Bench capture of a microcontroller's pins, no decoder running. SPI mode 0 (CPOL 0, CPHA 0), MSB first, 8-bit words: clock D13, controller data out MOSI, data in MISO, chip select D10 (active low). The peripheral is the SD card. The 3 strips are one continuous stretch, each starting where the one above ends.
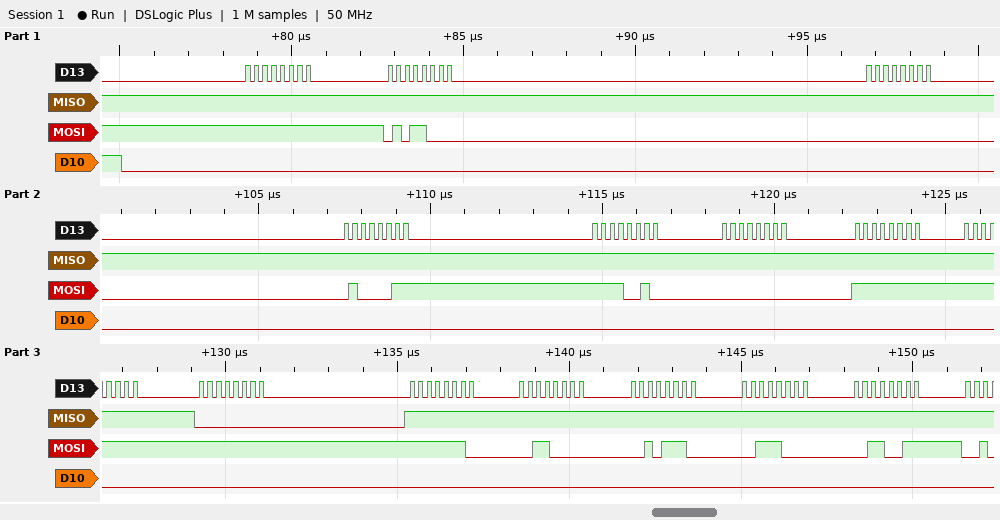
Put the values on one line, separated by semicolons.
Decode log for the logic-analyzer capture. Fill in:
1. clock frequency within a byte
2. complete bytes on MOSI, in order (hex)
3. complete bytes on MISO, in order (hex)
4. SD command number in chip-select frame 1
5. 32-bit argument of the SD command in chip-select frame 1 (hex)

4 MHz; FF 58 00 43 F2 00 FF FF FF FE 30 2E 38 33; FF FF FF FF FF FF FF FF 00 FF FF FF FF FF; CMD24; 0x0043F200
